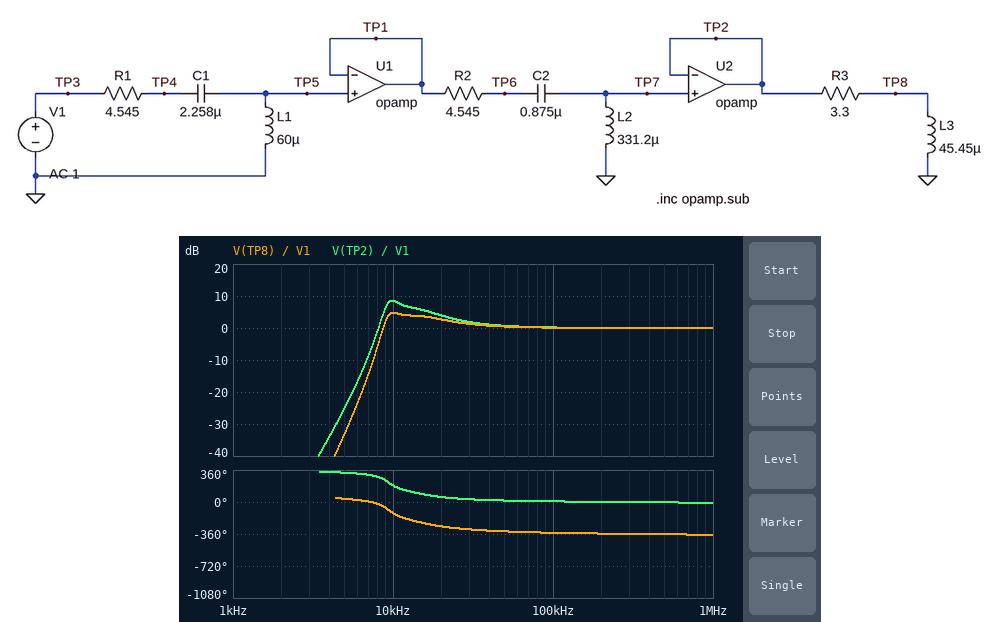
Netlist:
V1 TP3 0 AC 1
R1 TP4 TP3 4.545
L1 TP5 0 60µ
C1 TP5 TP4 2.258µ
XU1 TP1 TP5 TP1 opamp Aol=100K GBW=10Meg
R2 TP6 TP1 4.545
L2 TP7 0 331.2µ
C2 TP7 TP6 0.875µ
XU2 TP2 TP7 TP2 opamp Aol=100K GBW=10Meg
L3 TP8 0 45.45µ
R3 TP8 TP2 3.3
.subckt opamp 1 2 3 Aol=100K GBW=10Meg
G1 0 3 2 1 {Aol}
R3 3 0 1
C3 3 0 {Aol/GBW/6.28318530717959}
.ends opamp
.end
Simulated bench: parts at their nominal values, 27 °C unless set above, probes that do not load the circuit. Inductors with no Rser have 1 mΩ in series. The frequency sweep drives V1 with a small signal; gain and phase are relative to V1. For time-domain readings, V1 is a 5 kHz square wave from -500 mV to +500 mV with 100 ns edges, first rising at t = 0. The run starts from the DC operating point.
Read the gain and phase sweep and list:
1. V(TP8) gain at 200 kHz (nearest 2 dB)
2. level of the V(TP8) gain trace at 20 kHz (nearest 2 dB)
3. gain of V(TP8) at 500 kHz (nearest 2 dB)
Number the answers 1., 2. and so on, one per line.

1. 0 dB
2. 2 dB
3. 0 dB
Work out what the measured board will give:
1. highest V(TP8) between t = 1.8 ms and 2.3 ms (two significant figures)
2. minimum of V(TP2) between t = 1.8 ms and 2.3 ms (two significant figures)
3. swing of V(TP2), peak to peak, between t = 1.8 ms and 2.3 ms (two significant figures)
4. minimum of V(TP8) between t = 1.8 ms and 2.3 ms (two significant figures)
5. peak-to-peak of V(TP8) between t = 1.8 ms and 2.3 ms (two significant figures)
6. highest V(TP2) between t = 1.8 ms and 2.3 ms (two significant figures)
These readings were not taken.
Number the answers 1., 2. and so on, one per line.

1. 1.2 V
2. -1.2 V
3. 2.3 V
4. -1.2 V
5. 2.3 V
6. 1.2 V
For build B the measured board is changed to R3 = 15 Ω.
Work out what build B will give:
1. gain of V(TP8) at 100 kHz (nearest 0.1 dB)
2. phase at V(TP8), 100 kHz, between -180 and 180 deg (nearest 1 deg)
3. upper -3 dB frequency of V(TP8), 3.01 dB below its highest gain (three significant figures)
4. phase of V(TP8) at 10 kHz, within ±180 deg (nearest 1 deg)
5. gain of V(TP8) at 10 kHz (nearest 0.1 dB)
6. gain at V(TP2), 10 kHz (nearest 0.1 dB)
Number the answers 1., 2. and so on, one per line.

1. -0.9 dB
2. 35 deg
3. 6.51 MHz
4. -95 deg
5. -6.0 dB
6. 8.5 dB
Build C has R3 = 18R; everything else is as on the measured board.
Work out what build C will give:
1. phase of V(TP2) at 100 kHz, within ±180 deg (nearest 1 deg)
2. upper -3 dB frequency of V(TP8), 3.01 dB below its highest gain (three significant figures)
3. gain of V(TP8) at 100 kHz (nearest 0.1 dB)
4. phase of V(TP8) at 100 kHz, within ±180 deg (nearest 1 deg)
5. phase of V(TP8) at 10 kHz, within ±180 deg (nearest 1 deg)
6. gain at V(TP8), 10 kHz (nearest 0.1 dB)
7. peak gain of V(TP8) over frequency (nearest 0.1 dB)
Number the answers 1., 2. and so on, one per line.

1. 7 deg
2. 6.53 MHz
3. -1.3 dB
4. 39 deg
5. -93 deg
6. -7.6 dB
7. -0.1 dB
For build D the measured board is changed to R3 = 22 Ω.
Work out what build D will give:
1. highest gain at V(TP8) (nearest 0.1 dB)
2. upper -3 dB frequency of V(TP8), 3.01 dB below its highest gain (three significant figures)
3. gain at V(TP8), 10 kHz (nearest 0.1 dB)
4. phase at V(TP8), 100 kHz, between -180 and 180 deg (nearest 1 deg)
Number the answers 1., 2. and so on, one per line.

1. -0.1 dB
2. 6.55 MHz
3. -9.3 dB
4. 45 deg
